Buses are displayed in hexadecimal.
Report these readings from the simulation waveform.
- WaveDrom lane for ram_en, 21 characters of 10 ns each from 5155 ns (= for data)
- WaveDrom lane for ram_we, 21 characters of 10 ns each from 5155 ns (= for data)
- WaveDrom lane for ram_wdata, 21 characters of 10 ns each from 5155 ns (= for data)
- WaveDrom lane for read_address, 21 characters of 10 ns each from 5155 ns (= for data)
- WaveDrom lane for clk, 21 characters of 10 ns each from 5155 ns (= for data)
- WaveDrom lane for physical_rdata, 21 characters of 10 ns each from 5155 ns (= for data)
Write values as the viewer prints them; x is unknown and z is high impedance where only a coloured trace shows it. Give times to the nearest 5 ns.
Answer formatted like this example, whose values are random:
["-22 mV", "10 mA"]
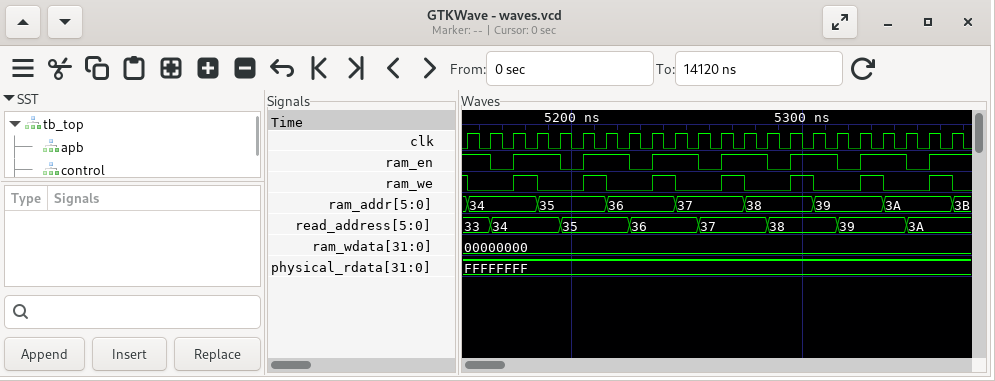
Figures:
["{name: 'ram_en', wave: '101.01.01.01.01.01.01'}", "{name: 'ram_we', wave: '0.10.10.10.10.10.10.1'}", "{name: 'ram_wdata', wave: '=....................', data: '00000000'}", "{name: 'read_address', wave: '==..=..=..=..=..=..=.', data: '33 34 35 36 37 38 39 3A'}", "{name: 'clk', wave: 'p....................'}", "{name: 'physical_rdata', wave: '=....................', data: 'FFFFFFFF'}"]
